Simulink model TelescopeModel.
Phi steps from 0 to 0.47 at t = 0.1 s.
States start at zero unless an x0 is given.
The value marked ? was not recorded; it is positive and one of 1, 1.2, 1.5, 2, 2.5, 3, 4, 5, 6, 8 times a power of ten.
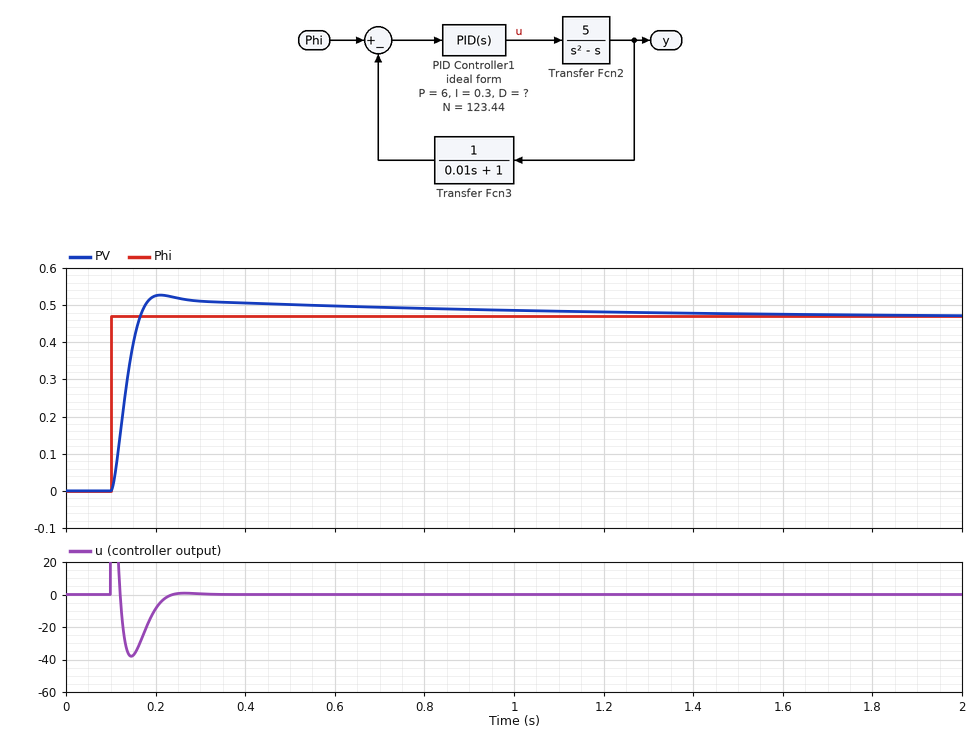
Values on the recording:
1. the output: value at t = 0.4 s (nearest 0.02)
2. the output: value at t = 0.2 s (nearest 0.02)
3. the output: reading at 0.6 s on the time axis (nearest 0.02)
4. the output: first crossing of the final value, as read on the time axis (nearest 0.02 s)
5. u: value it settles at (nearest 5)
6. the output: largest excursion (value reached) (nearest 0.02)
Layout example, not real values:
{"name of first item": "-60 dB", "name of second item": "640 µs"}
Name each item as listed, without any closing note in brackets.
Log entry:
{"the output: value at t = 0.4 s": "0.50", "the output: value at t = 0.2 s": "0.52", "the output: reading at 0.6 s on the time axis": "0.50", "the output: first crossing of the final value, as read on the time axis": "0.16 s", "u: value it settles at": "0", "the output: largest excursion (value reached)": "0.52"}
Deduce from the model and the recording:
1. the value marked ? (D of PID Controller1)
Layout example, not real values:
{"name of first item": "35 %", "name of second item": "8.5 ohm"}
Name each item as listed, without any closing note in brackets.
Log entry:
{"the value marked ?": "0.8"}
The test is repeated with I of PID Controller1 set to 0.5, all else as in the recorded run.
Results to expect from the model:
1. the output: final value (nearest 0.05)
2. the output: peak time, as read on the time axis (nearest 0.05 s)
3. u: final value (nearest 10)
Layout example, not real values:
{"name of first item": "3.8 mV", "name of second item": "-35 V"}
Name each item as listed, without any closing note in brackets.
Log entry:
{"the output: final value": "0.45", "the output: peak time, as read on the time axis": "0.20 s", "u: final value": "0"}
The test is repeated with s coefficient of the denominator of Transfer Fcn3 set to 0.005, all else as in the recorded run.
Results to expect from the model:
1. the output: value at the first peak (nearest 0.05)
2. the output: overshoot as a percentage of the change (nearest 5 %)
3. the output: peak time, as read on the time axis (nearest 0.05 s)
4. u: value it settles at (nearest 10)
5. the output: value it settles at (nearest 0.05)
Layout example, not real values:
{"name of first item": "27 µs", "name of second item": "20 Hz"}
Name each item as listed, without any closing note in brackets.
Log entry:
{"the output: value at the first peak": "0.50", "the output: overshoot as a percentage of the change": "10 %", "the output: peak time, as read on the time axis": "0.25 s", "u: value it settles at": "0", "the output: value it settles at": "0.45"}
